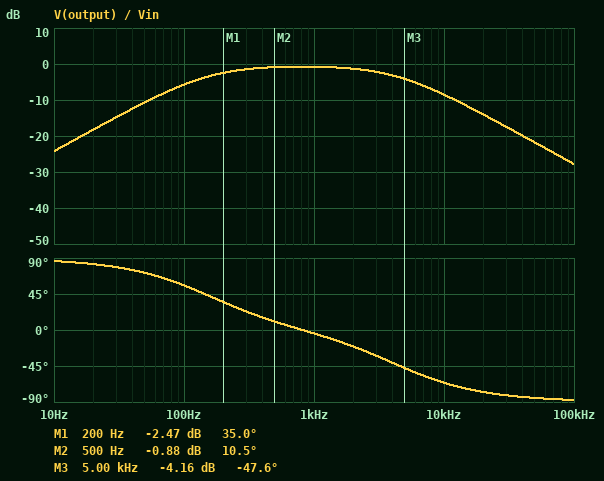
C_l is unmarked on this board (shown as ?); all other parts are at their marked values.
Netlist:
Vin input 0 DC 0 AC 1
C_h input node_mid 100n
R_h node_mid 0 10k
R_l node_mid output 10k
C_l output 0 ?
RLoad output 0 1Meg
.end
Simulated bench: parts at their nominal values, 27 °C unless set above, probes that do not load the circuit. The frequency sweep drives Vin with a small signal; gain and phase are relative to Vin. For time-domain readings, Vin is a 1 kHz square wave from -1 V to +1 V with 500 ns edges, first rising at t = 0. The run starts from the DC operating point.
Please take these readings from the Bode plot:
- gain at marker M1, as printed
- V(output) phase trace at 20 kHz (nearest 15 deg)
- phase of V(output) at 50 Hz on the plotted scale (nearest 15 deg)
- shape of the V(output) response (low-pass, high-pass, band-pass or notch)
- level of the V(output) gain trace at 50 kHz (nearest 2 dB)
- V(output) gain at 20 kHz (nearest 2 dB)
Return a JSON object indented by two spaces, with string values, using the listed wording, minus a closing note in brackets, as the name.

{
  "gain at marker M1, as printed": "-2.47 dB",
  "V(output) phase trace at 20 kHz": "-75 deg",
  "phase of V(output) at 50 Hz on the plotted scale": "75 deg",
  "shape of the V(output) response": "band-pass",
  "level of the V(output) gain trace at 50 kHz": "-22 dB",
  "V(output) gain at 20 kHz": "-14 dB"
}
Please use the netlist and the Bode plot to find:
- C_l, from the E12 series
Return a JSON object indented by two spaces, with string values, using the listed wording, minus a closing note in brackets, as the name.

{
  "C_l, from the E12 series": "3.9 nF"
}
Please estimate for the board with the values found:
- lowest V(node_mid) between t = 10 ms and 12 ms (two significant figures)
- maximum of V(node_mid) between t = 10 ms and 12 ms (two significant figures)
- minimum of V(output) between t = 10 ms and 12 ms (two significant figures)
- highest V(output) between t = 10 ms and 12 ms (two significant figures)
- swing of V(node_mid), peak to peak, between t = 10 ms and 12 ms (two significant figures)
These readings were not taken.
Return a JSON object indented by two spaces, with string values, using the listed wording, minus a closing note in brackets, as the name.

{
  "lowest V(node_mid) between t = 10 ms and 12 ms": "-1.3 V",
  "maximum of V(node_mid) between t = 10 ms and 12 ms": "1.3 V",
  "minimum of V(output) between t = 10 ms and 12 ms": "-1.0 V",
  "highest V(output) between t = 10 ms and 12 ms": "1.0 V",
  "swing of V(node_mid), peak to peak, between t = 10 ms and 12 ms": "2.5 V"
}
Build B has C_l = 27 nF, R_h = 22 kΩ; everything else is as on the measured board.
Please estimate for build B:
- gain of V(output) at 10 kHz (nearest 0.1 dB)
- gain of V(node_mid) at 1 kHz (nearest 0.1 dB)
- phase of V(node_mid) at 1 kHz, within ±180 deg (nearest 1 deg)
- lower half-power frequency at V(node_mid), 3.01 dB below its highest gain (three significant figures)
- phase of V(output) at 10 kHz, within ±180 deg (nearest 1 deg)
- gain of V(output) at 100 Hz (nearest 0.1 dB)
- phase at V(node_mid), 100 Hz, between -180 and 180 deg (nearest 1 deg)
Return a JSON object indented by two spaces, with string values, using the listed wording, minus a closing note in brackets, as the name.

{
  "gain of V(output) at 10 kHz": "-24.6 dB",
  "gain of V(node_mid) at 1 kHz": "-0.7 dB",
  "phase of V(node_mid) at 1 kHz, within ±180 deg": "10 deg",
  "lower half-power frequency at V(node_mid), 3.01 dB below its highest gain": "123 Hz",
  "phase of V(output) at 10 kHz, within ±180 deg": "-85 deg",
  "gain of V(output) at 100 Hz": "-3.6 dB",
  "phase at V(node_mid), 100 Hz, between -180 and 180 deg": "32 deg"
}
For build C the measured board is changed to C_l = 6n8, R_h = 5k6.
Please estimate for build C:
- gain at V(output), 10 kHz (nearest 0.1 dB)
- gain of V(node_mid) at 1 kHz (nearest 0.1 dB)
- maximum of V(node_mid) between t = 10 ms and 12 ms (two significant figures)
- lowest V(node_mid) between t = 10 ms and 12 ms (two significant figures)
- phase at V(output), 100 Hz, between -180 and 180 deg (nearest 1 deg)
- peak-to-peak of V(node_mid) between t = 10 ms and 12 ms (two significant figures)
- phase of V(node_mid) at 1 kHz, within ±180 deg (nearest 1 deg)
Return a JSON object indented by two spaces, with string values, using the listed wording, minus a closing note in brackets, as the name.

{
  "gain at V(output), 10 kHz": "-12.9 dB",
  "gain of V(node_mid) at 1 kHz": "-0.8 dB",
  "maximum of V(node_mid) between t = 10 ms and 12 ms": "1.4 V",
  "lowest V(node_mid) between t = 10 ms and 12 ms": "-1.4 V",
  "phase at V(output), 100 Hz, between -180 and 180 deg": "67 deg",
  "peak-to-peak of V(node_mid) between t = 10 ms and 12 ms": "2.9 V",
  "phase of V(node_mid) at 1 kHz, within ±180 deg": "16 deg"
}
